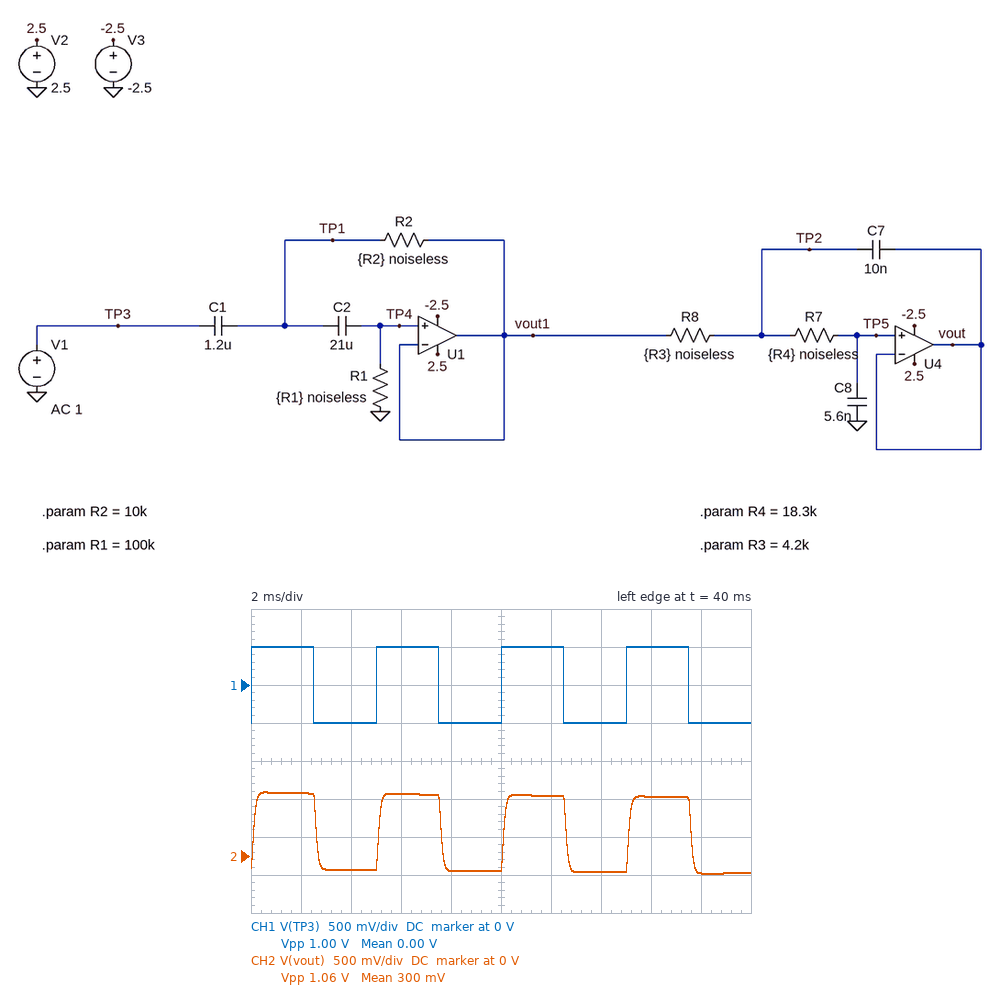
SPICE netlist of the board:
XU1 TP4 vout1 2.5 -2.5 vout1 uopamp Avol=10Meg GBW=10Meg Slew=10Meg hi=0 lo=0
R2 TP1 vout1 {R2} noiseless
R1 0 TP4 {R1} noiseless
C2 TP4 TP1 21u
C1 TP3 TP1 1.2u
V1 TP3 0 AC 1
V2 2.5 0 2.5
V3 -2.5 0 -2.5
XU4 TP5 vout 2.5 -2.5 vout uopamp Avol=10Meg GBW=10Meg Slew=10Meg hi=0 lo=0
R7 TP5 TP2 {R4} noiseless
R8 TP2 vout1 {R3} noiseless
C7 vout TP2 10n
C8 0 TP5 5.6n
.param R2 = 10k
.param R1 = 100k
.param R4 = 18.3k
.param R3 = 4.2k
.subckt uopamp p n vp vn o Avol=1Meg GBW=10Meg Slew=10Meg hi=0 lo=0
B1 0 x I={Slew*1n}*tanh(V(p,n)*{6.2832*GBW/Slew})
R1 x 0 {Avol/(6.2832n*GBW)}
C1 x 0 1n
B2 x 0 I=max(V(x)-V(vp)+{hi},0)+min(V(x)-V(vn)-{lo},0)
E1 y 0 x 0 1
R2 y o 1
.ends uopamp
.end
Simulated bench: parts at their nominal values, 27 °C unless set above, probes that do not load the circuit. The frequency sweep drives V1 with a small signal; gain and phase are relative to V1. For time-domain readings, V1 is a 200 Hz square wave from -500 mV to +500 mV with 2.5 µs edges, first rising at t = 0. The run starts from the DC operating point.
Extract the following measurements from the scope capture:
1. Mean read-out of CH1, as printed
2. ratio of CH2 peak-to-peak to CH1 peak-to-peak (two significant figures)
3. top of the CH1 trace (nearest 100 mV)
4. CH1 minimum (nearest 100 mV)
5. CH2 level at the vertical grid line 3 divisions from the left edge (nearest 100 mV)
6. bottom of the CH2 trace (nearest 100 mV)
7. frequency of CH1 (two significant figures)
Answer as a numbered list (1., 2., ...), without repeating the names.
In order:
1. 0.00 V
2. 1.1
3. 500 mV
4. -500 mV
5. 800 mV
6. -200 mV
7. 200 Hz
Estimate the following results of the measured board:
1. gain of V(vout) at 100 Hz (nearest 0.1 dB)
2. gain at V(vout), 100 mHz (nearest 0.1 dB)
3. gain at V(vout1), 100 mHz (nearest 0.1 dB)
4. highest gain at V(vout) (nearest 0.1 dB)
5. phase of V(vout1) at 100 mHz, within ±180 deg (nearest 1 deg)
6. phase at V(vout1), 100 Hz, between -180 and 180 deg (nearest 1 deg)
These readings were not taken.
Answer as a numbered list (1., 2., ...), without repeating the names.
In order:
1. 0 dB
2. -40.0 dB
3. -40.0 dB
4. 0 dB
5. 172 deg
6. 1 deg
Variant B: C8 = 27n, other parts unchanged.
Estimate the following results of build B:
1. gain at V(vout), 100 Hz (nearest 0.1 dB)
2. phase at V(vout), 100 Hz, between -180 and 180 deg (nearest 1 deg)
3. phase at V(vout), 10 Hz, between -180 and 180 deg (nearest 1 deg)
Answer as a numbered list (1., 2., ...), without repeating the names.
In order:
1. -0.5 dB
2. -20 deg
3. 6 deg
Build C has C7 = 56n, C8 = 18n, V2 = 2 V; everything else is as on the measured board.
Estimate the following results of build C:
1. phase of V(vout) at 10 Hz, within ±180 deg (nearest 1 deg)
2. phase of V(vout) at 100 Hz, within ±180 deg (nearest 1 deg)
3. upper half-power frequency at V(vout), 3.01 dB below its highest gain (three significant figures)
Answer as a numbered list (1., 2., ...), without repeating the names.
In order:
1. 7 deg
2. -14 deg
3. 555 Hz
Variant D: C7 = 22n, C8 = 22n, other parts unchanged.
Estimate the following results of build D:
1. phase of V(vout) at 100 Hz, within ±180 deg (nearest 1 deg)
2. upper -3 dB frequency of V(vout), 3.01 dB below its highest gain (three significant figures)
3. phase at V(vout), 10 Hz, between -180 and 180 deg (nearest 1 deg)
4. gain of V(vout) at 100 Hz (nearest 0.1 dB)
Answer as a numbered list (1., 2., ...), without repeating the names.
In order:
1. -17 deg
2. 377 Hz
3. 6 deg
4. -0.3 dB
